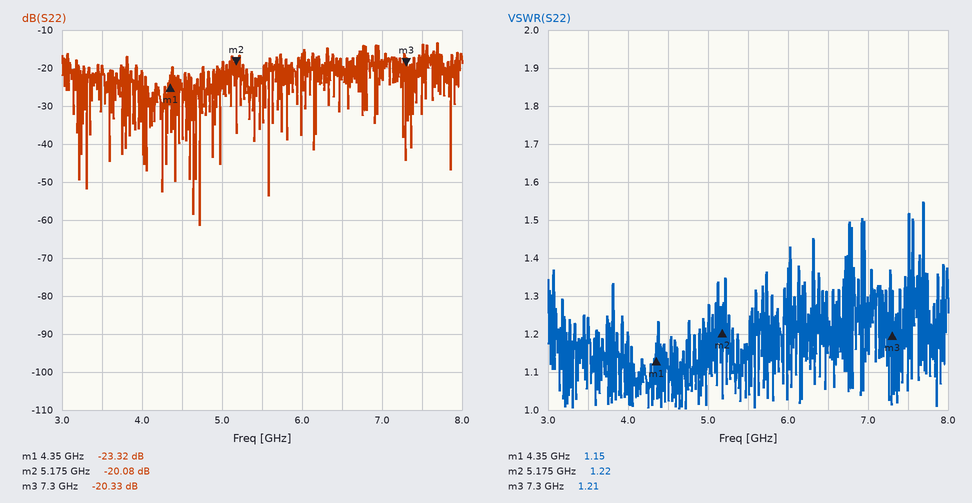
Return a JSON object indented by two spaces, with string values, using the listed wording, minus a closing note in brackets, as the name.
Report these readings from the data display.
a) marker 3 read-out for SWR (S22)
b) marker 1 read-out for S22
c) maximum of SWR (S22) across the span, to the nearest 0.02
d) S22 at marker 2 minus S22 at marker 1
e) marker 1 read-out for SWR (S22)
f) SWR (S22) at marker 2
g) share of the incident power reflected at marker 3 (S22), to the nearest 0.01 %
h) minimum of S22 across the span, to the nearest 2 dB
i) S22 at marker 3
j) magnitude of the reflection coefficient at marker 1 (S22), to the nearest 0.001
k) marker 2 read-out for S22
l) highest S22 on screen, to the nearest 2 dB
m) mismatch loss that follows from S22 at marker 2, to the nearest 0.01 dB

{
  "marker 3 read-out for SWR": "1.21",
  "marker 1 read-out for S22": "-23.32 dB",
  "maximum of SWR (S22) across the span, to the nearest 0.02": "1.54",
  "S22 at marker 2 minus S22 at marker 1": "3.24 dB",
  "marker 1 read-out for SWR": "1.15",
  "SWR (S22) at marker 2": "1.22",
  "share of the incident power reflected at marker 3 (S22), to the nearest 0.01 %": "0.93 %",
  "minimum of S22 across the span, to the nearest 2 dB": "-62 dB",
  "S22 at marker 3": "-20.33 dB",
  "magnitude of the reflection coefficient at marker 1 (S22), to the nearest 0.001": "0.068",
  "marker 2 read-out for S22": "-20.08 dB",
  "highest S22 on screen, to the nearest 2 dB": "-14 dB",
  "mismatch loss that follows from S22 at marker 2, to the nearest 0.01 dB": "0.04 dB"
}
